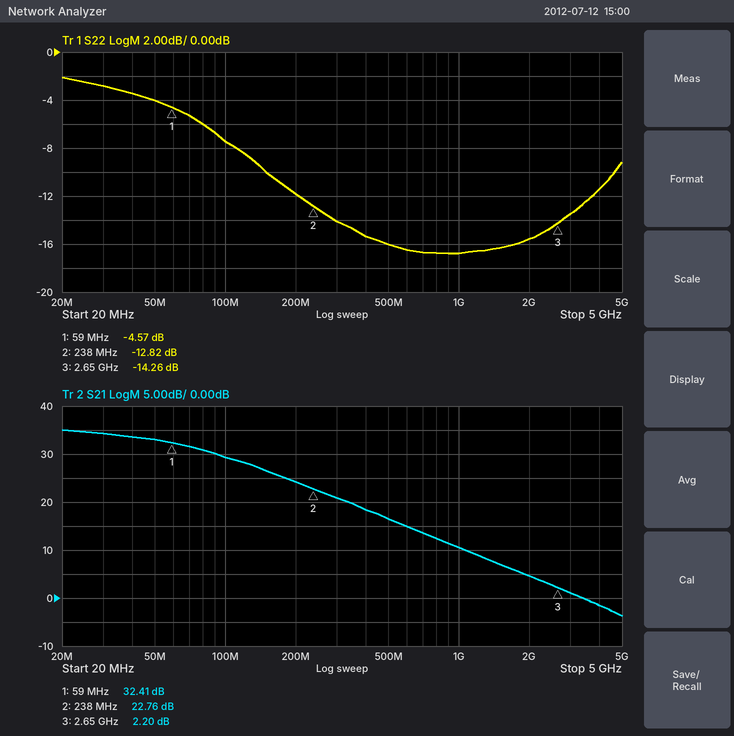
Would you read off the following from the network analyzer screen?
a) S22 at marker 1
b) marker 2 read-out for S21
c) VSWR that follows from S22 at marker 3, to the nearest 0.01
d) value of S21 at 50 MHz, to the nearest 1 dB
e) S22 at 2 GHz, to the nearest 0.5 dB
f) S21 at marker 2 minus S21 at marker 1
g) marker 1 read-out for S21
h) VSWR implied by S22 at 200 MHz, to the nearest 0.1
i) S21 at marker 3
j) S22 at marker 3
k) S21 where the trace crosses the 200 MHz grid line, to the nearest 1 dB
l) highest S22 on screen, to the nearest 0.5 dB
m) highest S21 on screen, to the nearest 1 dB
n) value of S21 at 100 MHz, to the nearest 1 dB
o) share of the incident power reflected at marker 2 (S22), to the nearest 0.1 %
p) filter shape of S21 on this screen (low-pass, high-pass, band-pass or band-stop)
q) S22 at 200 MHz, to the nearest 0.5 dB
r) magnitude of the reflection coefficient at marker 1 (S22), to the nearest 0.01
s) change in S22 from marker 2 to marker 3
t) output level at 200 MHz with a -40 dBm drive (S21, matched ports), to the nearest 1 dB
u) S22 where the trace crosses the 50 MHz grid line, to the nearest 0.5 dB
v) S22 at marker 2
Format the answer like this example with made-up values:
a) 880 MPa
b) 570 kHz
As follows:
a) -4.57 dB
b) 22.76 dB
c) 1.48
d) 33 dB
e) -15.5 dB
f) -9.65 dB
g) 32.41 dB
h) 1.7
i) 2.20 dB
j) -14.26 dB
k) 24 dB
l) -2.0 dB
m) 35 dB
n) 29 dB
o) 5.2 %
p) low-pass
q) -12.0 dB
r) 0.59
s) -1.44 dB
t) -16 dBm
u) -4.0 dB
v) -12.82 dB
